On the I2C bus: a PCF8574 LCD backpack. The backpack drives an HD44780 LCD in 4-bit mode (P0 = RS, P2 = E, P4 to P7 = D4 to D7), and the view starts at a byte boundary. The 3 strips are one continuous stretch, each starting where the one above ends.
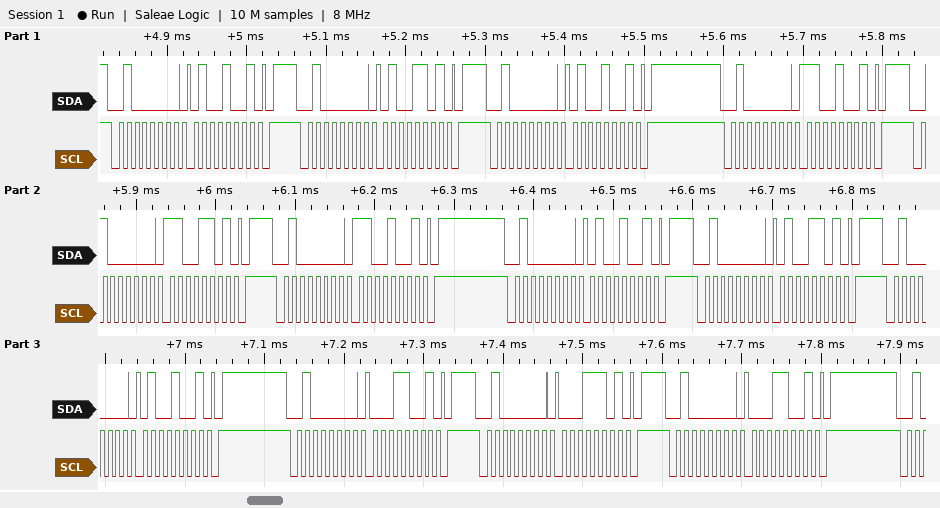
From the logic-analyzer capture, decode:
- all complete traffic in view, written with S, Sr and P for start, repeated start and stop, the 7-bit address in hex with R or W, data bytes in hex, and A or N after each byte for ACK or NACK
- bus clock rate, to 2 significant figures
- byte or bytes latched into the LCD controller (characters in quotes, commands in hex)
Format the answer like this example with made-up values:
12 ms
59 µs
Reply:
S 20W A 49 A P S 20W A 4D A P S 20W A 49 A P S 20W A C9 A P S 20W A CD A P S 20W A C9 A P S 20W A 49 A P S 20W A 4D A P S 20W A 49 A P S 20W A 19 A P S 20W A 1D A P S 20W A 19 A P
100 kHz
'L' 'A'
